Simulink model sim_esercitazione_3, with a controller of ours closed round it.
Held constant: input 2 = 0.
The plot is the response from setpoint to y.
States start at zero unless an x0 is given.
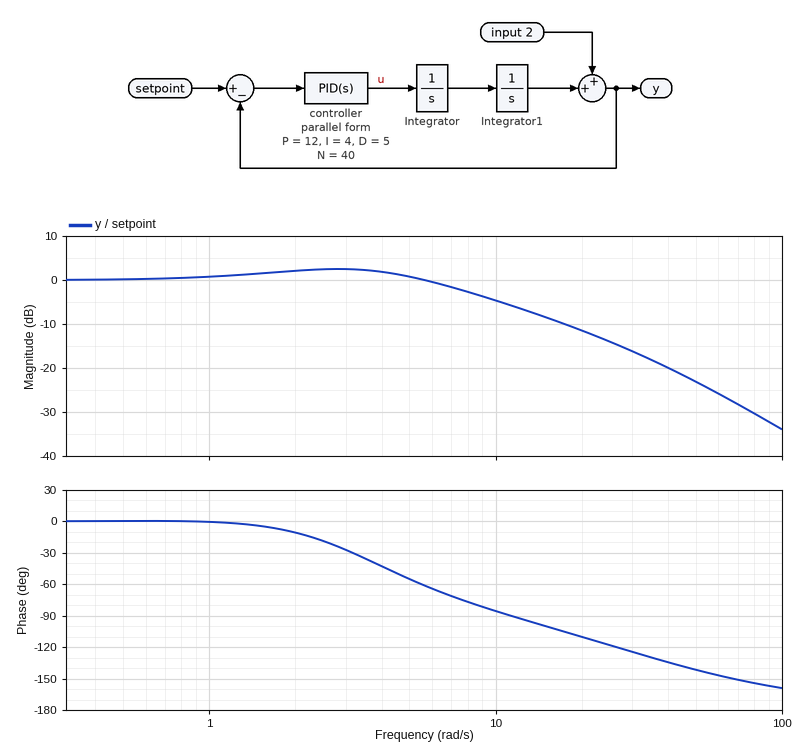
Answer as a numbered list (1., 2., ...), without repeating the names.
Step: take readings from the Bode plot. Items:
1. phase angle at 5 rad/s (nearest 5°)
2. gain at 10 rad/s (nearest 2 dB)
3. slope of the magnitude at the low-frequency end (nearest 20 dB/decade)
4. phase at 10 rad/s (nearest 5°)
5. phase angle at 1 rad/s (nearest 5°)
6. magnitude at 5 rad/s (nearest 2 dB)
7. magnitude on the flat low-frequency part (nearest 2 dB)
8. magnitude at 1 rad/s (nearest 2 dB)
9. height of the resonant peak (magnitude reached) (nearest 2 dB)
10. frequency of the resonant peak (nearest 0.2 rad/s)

1. -55°
2. -4 dB
3. 0 dB/decade
4. -85°
5. 0°
6. 0 dB
7. 0 dB
8. 0 dB
9. 2 dB
10. 2.8 rad/s
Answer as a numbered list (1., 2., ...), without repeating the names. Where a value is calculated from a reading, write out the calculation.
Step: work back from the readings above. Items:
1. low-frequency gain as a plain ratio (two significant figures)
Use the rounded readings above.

1. 10^(0 / 20) = 1.0
